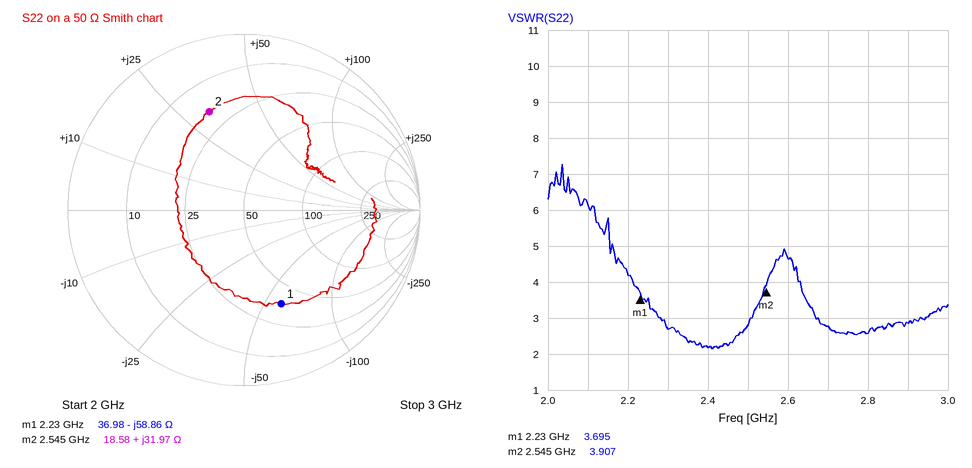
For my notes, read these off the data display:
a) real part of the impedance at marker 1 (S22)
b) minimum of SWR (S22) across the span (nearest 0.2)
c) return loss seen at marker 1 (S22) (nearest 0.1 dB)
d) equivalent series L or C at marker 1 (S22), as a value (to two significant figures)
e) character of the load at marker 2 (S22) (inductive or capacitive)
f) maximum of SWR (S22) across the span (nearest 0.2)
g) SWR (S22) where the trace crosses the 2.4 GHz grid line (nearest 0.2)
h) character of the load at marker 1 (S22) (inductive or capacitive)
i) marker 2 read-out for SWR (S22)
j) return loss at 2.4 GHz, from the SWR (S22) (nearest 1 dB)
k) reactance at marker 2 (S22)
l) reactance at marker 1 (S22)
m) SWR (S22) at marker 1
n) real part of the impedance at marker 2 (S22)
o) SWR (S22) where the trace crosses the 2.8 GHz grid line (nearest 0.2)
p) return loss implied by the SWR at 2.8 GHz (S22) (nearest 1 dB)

36.98 Ω
2.2
4.8 dB
1.2 pF
inductive
7.2
2.2
capacitive
3.907
9 dB
+31.97 Ω
-58.86 Ω
3.695
18.58 Ω
2.6
7 dB
